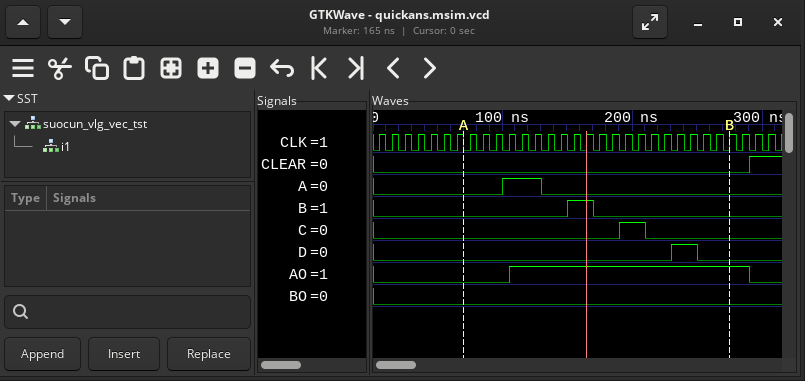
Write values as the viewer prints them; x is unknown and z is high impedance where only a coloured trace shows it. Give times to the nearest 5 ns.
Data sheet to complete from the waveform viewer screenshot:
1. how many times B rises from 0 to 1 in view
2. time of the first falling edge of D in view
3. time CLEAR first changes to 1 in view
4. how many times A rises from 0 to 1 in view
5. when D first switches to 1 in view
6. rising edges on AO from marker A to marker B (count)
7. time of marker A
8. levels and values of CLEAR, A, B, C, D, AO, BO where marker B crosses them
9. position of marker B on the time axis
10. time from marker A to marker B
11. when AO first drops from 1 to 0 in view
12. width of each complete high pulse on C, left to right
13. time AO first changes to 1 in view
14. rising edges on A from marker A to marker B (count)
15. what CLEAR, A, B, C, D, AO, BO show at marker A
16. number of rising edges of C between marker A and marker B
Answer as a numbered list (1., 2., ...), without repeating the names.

1. 1
2. 250 ns
3. 290 ns
4. 1
5. 230 ns
6. 1
7. 70 ns
8. CLEAR=0, A=0, B=0, C=0, D=0, AO=1, BO=0
9. 275 ns
10. 205 ns
11. 290 ns
12. 20 ns
13. 105 ns
14. 1
15. CLEAR=0, A=0, B=0, C=0, D=0, AO=0, BO=0
16. 1
